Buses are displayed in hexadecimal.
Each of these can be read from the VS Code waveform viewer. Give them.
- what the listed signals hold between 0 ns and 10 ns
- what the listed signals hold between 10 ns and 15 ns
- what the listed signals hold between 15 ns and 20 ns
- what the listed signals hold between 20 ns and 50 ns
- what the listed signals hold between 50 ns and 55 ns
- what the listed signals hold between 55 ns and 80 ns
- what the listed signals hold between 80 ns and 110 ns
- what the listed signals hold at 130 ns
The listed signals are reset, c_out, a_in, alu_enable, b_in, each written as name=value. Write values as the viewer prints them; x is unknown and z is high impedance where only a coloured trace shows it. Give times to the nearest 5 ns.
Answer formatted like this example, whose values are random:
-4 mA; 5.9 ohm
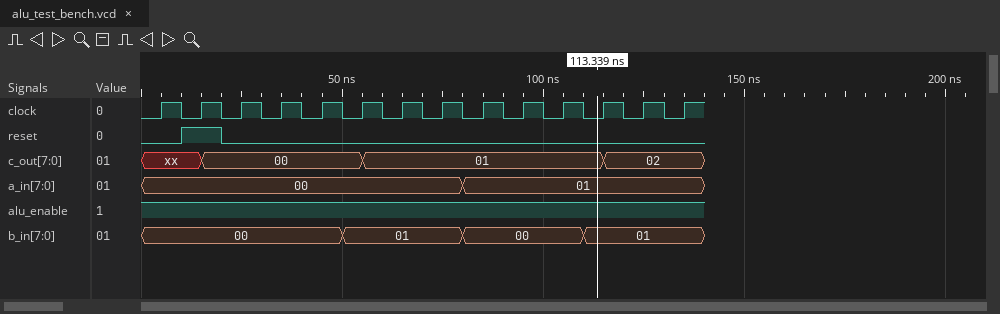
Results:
reset=0, c_out=xx, a_in=00, alu_enable=1, b_in=00; reset=1, c_out=xx, a_in=00, alu_enable=1, b_in=00; reset=1, c_out=00, a_in=00, alu_enable=1, b_in=00; reset=0, c_out=00, a_in=00, alu_enable=1, b_in=00; reset=0, c_out=00, a_in=00, alu_enable=1, b_in=01; reset=0, c_out=01, a_in=00, alu_enable=1, b_in=01; reset=0, c_out=01, a_in=01, alu_enable=1, b_in=00; reset=0, c_out=02, a_in=01, alu_enable=1, b_in=01
